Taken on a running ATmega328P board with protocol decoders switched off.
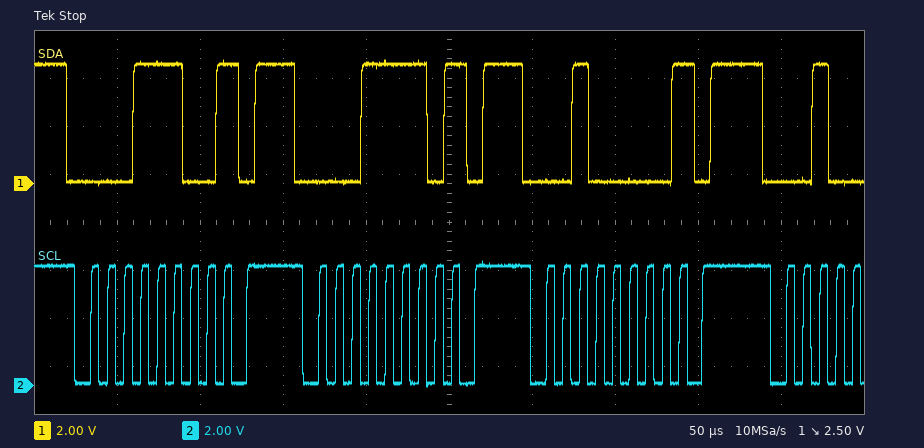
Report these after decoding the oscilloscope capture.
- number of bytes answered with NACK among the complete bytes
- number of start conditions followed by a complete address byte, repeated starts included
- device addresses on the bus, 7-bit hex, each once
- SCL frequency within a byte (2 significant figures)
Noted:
3
3
0x0E 0x0F 0x10
100 kHz
